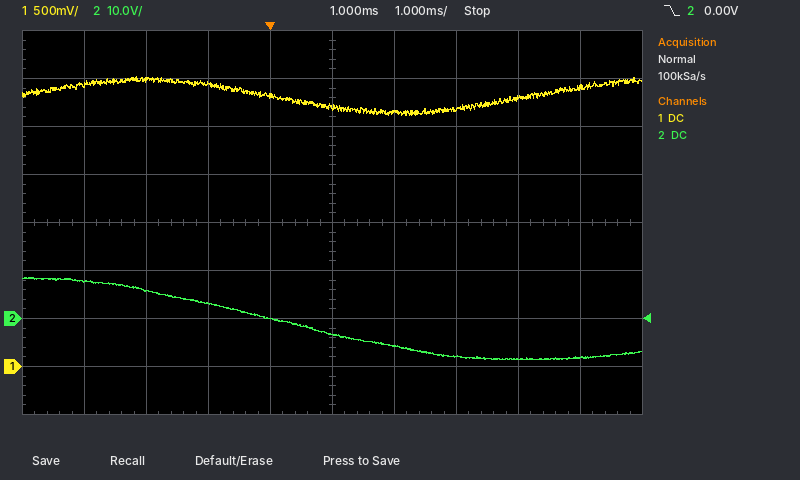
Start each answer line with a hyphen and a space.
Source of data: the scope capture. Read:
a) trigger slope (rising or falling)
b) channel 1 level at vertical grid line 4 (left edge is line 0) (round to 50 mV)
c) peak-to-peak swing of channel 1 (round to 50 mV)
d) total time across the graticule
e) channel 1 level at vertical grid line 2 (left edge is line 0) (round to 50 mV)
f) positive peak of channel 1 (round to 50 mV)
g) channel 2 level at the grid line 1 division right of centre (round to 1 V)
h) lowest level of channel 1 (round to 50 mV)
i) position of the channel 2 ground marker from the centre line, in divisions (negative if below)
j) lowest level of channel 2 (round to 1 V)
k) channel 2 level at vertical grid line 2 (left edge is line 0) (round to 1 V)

- falling
- 2.80 V
- 400 mV
- 10 ms
- 3.00 V
- 3.00 V
- -6 V
- 2.60 V
- -2.0 div
- -9 V
- 6 V
